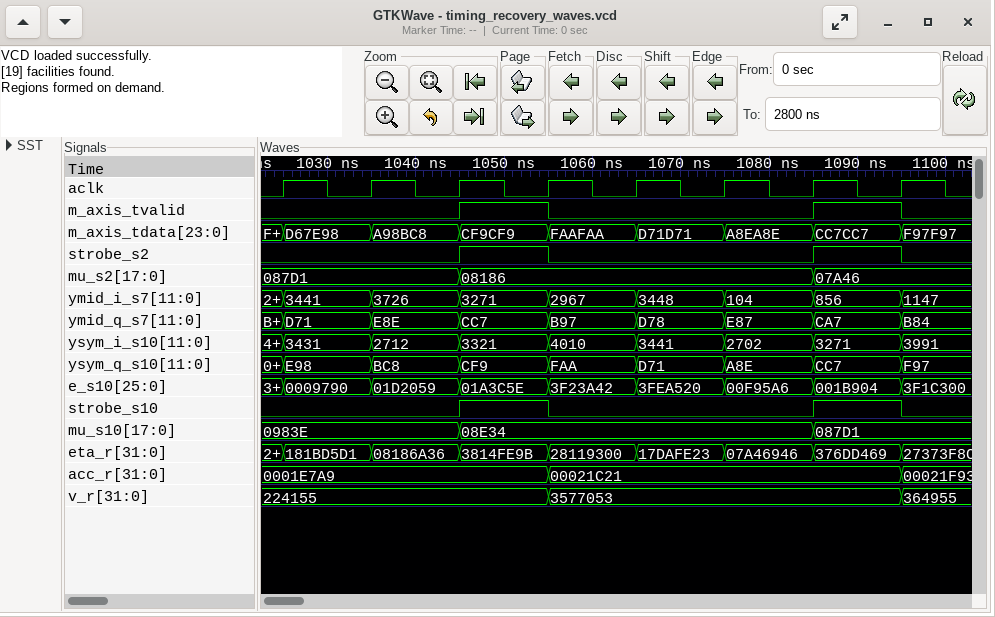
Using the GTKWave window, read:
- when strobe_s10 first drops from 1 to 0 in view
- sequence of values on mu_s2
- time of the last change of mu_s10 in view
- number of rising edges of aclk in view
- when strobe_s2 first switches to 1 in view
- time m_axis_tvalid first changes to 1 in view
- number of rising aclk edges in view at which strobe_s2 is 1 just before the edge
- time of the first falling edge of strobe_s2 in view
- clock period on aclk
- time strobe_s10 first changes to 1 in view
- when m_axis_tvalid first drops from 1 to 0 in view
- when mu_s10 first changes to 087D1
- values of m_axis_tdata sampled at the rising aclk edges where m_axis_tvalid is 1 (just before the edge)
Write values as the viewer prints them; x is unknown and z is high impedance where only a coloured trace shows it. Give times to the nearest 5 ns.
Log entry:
1055 ns
087D1, 08186, 07A46
1085 ns
8
1045 ns
1045 ns
2
1055 ns
10 ns
1045 ns
1055 ns
1085 ns
CF9CF9, CC7CC7
